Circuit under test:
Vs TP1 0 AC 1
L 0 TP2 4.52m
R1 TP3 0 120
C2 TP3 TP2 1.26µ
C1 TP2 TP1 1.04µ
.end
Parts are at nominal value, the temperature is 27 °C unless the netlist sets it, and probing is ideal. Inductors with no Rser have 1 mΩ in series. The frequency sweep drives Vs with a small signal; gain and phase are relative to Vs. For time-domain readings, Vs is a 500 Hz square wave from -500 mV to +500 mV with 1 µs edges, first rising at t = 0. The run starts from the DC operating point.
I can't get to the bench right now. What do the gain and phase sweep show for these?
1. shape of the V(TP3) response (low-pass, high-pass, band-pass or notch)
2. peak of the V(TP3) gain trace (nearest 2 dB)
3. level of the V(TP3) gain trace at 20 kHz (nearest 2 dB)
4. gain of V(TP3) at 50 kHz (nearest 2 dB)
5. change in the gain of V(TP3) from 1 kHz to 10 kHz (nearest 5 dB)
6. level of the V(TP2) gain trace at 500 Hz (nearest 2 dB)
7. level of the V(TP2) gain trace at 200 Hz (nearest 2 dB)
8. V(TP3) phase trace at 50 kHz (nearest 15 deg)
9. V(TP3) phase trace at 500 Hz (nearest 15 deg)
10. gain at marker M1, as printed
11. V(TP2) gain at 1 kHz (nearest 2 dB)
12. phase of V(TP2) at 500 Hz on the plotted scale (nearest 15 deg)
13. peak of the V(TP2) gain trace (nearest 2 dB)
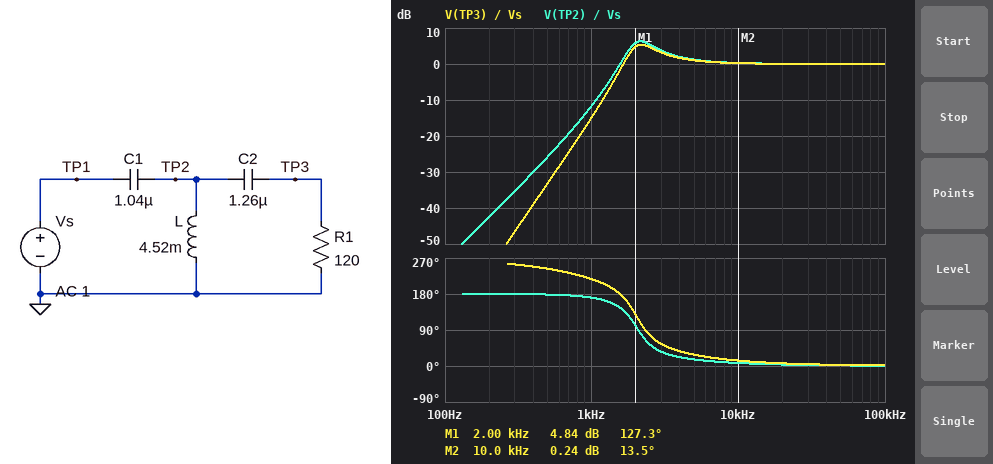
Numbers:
high-pass
6 dB
0 dB
0 dB
15 dB
-26 dB
-42 dB
0 deg
240 deg
4.84 dB
-12 dB
180 deg
6 dB
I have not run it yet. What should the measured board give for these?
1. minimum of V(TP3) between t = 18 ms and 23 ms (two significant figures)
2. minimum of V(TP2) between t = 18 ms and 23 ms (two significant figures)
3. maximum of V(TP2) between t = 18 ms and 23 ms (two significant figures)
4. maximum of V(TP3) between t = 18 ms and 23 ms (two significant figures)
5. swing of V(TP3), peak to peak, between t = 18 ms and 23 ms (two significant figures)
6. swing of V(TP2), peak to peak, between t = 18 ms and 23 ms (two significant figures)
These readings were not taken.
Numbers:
-960 mV
-950 mV
950 mV
960 mV
1.9 V
1.9 V
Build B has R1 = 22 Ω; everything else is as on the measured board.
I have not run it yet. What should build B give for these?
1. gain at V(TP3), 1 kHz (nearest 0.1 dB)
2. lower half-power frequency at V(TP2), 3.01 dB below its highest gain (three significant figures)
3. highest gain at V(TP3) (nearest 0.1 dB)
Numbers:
-25.5 dB
1.48 kHz
0 dB
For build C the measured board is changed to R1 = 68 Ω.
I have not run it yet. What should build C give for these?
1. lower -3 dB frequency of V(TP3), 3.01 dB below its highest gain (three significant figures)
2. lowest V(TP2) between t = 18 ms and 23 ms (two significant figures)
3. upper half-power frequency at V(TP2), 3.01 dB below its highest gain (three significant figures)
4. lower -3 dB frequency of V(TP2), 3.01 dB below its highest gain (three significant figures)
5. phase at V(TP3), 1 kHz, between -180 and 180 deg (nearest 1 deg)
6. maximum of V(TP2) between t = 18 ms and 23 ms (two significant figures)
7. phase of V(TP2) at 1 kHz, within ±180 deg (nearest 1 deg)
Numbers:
1.56 kHz
-980 mV
2.68 kHz
1.52 kHz
-127 deg
980 mV
172 deg
